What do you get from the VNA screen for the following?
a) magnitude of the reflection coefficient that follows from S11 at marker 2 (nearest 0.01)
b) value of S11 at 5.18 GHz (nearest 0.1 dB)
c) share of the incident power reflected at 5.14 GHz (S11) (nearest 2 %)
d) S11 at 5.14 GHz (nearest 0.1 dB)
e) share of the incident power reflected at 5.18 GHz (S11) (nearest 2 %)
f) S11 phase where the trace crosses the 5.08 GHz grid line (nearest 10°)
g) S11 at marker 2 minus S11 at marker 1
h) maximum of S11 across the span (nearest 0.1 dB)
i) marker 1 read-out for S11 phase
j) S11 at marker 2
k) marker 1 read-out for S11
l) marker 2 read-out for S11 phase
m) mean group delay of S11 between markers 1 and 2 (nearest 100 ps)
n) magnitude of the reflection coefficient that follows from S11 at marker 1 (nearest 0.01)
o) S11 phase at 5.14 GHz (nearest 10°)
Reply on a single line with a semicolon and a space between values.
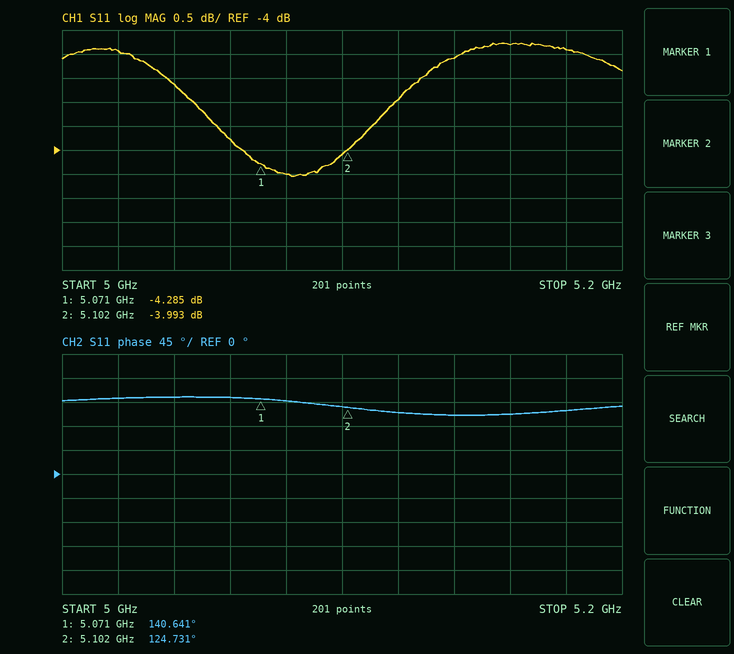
0.63; -1.9 dB; 62 %; -2.1 dB; 64 %; 140°; 0.292 dB; -1.8 dB; 140.641°; -3.993 dB; -4.285 dB; 124.731°; 1.4 ns; 0.61; 110°
